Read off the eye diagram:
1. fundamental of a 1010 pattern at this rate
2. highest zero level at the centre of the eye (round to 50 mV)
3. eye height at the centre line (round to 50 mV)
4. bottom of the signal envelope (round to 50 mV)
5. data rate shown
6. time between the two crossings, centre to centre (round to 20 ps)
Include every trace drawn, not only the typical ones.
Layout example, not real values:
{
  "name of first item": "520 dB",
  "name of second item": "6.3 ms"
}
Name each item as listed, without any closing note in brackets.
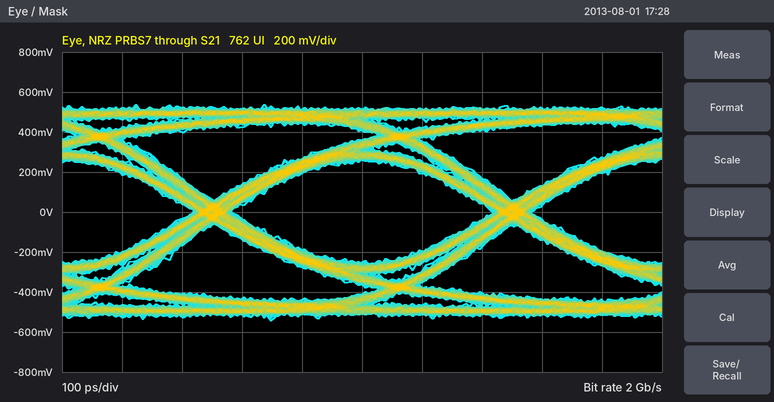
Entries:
{
  "fundamental of a 1010 pattern at this rate": "1 GHz",
  "highest zero level at the centre of the eye": "-250 mV",
  "eye height at the centre line": "500 mV",
  "bottom of the signal envelope": "-550 mV",
  "data rate shown": "2 Gb/s",
  "time between the two crossings, centre to centre": "500 ps"
}
